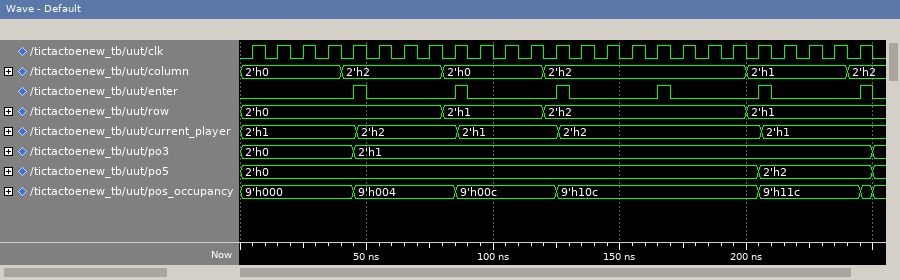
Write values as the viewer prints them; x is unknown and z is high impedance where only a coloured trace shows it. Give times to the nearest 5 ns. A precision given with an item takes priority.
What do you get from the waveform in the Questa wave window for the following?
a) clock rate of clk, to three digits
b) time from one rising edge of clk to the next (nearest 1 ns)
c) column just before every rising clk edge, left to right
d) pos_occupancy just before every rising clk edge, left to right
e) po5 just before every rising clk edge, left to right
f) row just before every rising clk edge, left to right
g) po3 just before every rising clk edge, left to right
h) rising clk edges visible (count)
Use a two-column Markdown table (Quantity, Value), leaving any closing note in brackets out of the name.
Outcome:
| Quantity | Value |
|---|---|
| clock rate of clk, to three digits | 100 MHz |
| time from one rising edge of clk to the next | 10 ns |
| column just before every rising clk edge, left to right | 2'h0, 2'h0, 2'h0, 2'h0, 2'h2, 2'h2, 2'h2, 2'h2, 2'h0, 2'h0, 2'h0, 2'h0, 2'h2, 2'h2, 2'h2, 2'h2, 2'h2, 2'h2, 2'h2, 2'h2, 2'h1, 2'h1, 2'h1, 2'h1, 2'h2 |
| pos_occupancy just before every rising clk edge, left to right | 9'h000, 9'h000, 9'h000, 9'h000, 9'h000, 9'h004, 9'h004, 9'h004, 9'h004, 9'h00c, 9'h00c, 9'h00c, 9'h00c, 9'h10c, 9'h10c, 9'h10c, 9'h10c, 9'h10c, 9'h10c, 9'h10c, 9'h10c, 9'h11c, 9'h11c, 9'h11c, 9'h11c |
| po5 just before every rising clk edge, left to right | 2'h0, 2'h0, 2'h0, 2'h0, 2'h0, 2'h0, 2'h0, 2'h0, 2'h0, 2'h0, 2'h0, 2'h0, 2'h0, 2'h0, 2'h0, 2'h0, 2'h0, 2'h0, 2'h0, 2'h0, 2'h0, 2'h2, 2'h2, 2'h2, 2'h2 |
| row just before every rising clk edge, left to right | 2'h0, 2'h0, 2'h0, 2'h0, 2'h0, 2'h0, 2'h0, 2'h0, 2'h1, 2'h1, 2'h1, 2'h1, 2'h2, 2'h2, 2'h2, 2'h2, 2'h2, 2'h2, 2'h2, 2'h2, 2'h1, 2'h1, 2'h1, 2'h1, 2'h1 |
| po3 just before every rising clk edge, left to right | 2'h0, 2'h0, 2'h0, 2'h0, 2'h0, 2'h1, 2'h1, 2'h1, 2'h1, 2'h1, 2'h1, 2'h1, 2'h1, 2'h1, 2'h1, 2'h1, 2'h1, 2'h1, 2'h1, 2'h1, 2'h1, 2'h1, 2'h1, 2'h1, 2'h1 |
| rising clk edges visible | 25 |
